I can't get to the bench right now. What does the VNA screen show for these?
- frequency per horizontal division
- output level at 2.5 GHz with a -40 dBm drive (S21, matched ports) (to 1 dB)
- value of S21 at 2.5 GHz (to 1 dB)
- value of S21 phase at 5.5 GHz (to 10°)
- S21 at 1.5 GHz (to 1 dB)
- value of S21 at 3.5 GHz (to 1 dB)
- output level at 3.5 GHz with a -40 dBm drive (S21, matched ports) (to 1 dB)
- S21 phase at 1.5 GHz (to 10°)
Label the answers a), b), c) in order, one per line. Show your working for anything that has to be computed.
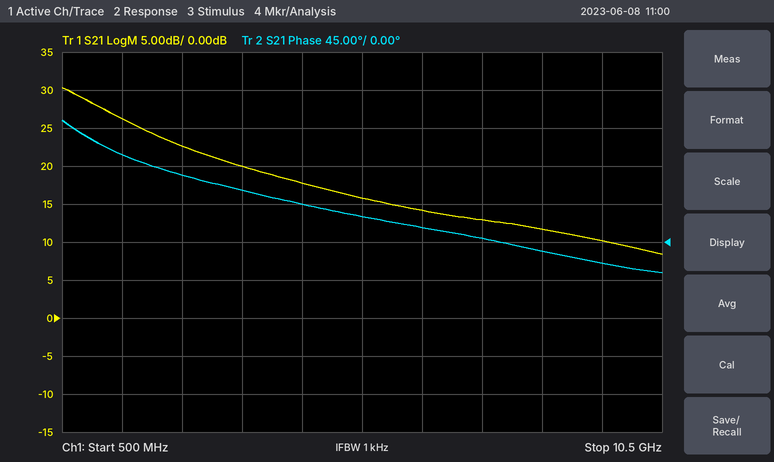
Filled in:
a) 1 GHz
b) -40 dBm + (23 dB) = -17 dBm
c) 23 dB
d) 30°
e) 26 dB
f) 20 dB
g) -40 dBm + (20 dB) = -20 dBm
h) 100°
